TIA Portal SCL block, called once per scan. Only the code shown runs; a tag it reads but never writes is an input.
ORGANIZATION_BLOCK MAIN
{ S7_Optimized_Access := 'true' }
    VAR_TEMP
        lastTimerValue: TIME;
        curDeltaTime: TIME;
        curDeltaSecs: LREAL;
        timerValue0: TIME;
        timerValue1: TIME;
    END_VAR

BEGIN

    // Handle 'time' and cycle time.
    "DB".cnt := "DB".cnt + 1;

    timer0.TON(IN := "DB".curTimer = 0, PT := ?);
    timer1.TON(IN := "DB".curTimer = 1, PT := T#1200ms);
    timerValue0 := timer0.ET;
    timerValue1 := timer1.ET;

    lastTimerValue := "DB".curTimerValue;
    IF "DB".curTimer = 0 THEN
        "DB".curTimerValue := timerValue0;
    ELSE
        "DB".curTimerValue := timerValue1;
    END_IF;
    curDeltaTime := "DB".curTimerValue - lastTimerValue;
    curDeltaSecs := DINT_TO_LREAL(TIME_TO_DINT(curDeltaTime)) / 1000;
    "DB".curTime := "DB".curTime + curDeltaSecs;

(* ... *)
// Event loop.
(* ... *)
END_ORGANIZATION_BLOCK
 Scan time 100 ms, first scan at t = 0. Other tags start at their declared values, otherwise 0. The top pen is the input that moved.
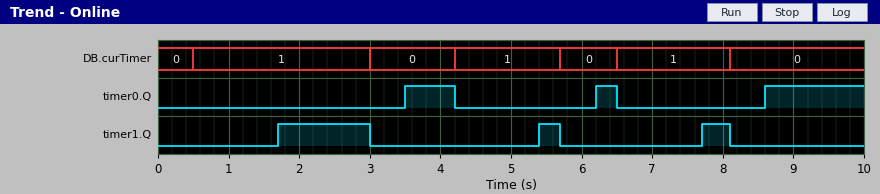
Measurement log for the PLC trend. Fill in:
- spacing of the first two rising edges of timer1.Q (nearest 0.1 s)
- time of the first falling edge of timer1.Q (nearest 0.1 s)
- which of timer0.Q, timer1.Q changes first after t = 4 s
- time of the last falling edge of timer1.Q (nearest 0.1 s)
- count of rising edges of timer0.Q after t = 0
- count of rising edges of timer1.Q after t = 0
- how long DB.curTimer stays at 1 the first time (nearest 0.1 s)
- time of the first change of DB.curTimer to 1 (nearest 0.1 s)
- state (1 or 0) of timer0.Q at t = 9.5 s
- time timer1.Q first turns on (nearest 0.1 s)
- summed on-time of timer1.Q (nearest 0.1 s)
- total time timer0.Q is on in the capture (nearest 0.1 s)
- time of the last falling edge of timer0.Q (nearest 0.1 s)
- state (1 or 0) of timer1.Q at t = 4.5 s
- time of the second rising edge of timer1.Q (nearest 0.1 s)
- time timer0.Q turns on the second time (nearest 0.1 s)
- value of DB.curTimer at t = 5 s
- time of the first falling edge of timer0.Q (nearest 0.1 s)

3.7 s
3.0 s
timer0.Q
8.1 s
3
3
2.5 s
0.5 s
1
1.7 s
2.0 s
2.4 s
6.5 s
0
5.4 s
6.2 s
1
4.2 s
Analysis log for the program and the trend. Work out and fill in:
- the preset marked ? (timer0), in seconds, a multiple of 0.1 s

0.5 s
